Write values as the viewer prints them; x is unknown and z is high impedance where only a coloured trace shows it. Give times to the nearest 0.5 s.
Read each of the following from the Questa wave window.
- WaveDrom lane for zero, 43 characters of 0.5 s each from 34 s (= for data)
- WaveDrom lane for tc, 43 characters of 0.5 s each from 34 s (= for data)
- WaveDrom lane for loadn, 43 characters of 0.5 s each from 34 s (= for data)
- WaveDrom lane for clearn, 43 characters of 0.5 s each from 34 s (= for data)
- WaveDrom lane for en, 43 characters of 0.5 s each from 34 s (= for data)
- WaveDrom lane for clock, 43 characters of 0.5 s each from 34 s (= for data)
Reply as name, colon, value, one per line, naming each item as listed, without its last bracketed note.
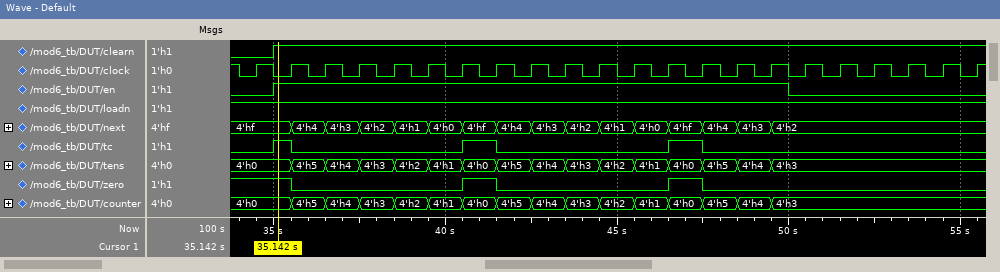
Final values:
WaveDrom lane for zero, 43 characters of 0.5 s each from 34 s: {name: 'zero', wave: '1..0.........1.0.........1.0...............'}
WaveDrom lane for tc, 43 characters of 0.5 s each from 34 s: {name: 'tc', wave: '0.10.........1.0.........1.0...............'}
WaveDrom lane for loadn, 43 characters of 0.5 s each from 34 s: {name: 'loadn', wave: '1..........................................'}
WaveDrom lane for clearn, 43 characters of 0.5 s each from 34 s: {name: 'clearn', wave: '0.1........................................'}
WaveDrom lane for en, 43 characters of 0.5 s each from 34 s: {name: 'en', wave: '0.1.............................0..........'}
WaveDrom lane for clock, 43 characters of 0.5 s each from 34 s: {name: 'clock', wave: '0101010101010101010101010101010101010101010'}
